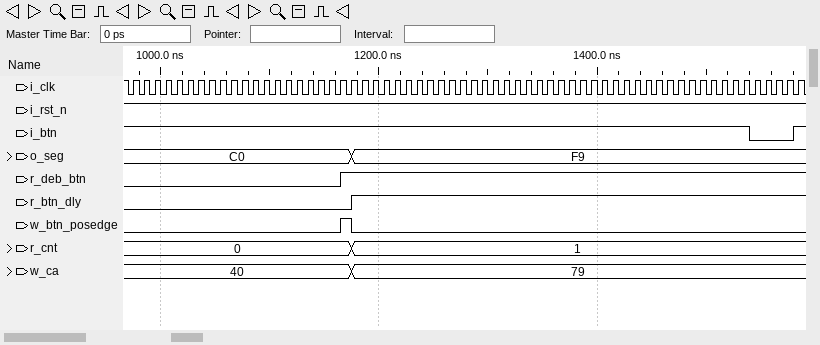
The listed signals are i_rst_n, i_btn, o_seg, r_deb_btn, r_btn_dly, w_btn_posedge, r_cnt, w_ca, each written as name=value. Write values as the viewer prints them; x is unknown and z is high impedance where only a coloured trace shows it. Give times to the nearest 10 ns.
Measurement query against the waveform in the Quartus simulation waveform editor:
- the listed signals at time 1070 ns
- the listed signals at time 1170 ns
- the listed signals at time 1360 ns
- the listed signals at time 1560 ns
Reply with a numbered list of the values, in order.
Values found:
1. i_rst_n=1, i_btn=1, o_seg=C0, r_deb_btn=0, r_btn_dly=0, w_btn_posedge=0, r_cnt=0, w_ca=40
2. i_rst_n=1, i_btn=1, o_seg=C0, r_deb_btn=1, r_btn_dly=0, w_btn_posedge=1, r_cnt=0, w_ca=40
3. i_rst_n=1, i_btn=1, o_seg=F9, r_deb_btn=1, r_btn_dly=1, w_btn_posedge=0, r_cnt=1, w_ca=79
4. i_rst_n=1, i_btn=0, o_seg=F9, r_deb_btn=1, r_btn_dly=1, w_btn_posedge=0, r_cnt=1, w_ca=79
